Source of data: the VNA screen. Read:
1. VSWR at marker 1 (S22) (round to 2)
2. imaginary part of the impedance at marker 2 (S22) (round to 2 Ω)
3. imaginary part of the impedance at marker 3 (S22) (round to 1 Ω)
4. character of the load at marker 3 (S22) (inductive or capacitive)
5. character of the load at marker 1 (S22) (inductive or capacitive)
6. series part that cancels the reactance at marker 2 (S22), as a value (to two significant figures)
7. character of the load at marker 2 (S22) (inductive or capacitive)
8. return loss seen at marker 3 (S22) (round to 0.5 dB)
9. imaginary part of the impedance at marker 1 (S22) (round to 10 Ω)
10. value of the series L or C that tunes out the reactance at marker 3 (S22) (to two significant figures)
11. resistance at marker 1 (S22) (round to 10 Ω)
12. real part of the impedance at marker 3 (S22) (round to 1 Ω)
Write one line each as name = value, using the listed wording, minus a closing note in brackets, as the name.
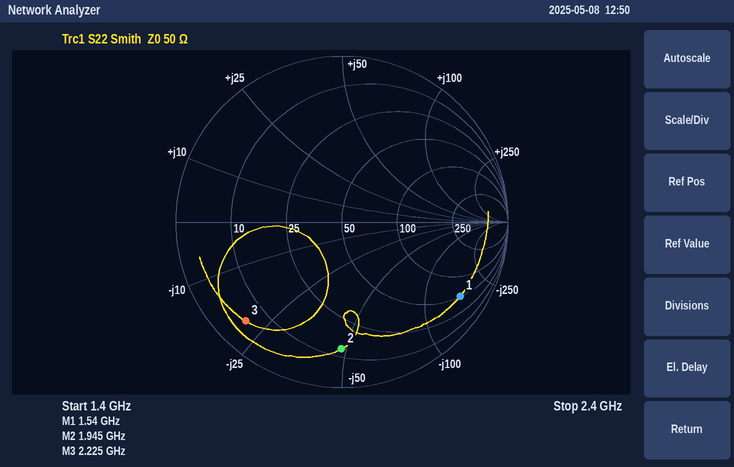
VSWR at marker 1 (S22) = 12
imaginary part of the impedance at marker 2 (S22) = -48 Ω
imaginary part of the impedance at marker 3 (S22) = -21 Ω
character of the load at marker 3 (S22) = capacitive
character of the load at marker 1 (S22) = capacitive
series part that cancels the reactance at marker 2 (S22), as a value = 3.9 nH
character of the load at marker 2 (S22) = capacitive
return loss seen at marker 3 (S22) = 1.5 dB
imaginary part of the impedance at marker 1 (S22) = -160 Ω
value of the series L or C that tunes out the reactance at marker 3 (S22) = 1.5 nH
resistance at marker 1 (S22) = 50 Ω
real part of the impedance at marker 3 (S22) = 5 Ω
